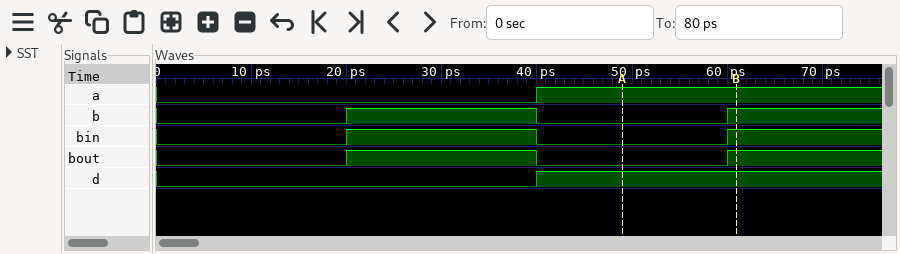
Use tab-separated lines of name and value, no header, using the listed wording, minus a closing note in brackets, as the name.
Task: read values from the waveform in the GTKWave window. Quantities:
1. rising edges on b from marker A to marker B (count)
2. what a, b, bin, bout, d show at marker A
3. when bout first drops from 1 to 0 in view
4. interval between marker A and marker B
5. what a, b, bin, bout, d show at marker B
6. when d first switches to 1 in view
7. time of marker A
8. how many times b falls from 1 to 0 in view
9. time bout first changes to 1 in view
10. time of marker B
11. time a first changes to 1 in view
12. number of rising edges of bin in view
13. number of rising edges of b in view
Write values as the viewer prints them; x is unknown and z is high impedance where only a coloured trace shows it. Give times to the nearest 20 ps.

rising edges on b from marker A to marker B	1
what a, b, bin, bout, d show at marker A	a=1, b=0, bin=0, bout=0, d=1
when bout first drops from 1 to 0 in view	40 ps
interval between marker A and marker B	20 ps
what a, b, bin, bout, d show at marker B	a=1, b=1, bin=1, bout=1, d=1
when d first switches to 1 in view	40 ps
time of marker A	40 ps
how many times b falls from 1 to 0 in view	1
time bout first changes to 1 in view	20 ps
time of marker B	60 ps
time a first changes to 1 in view	40 ps
number of rising edges of bin in view	2
number of rising edges of b in view	2
